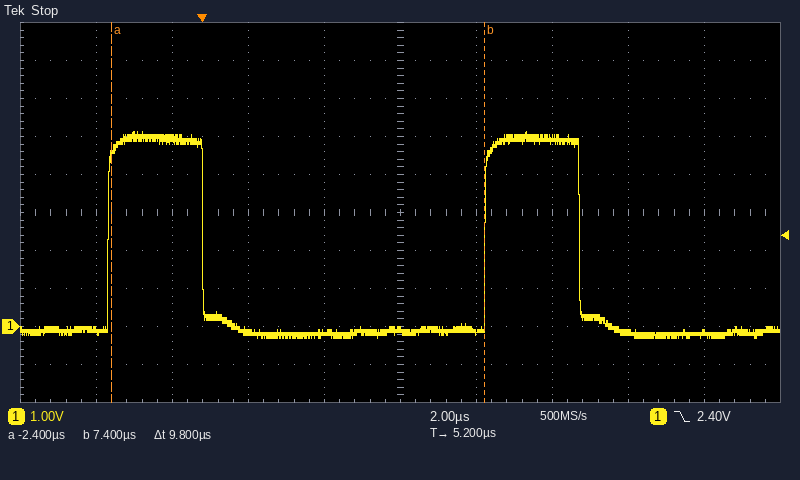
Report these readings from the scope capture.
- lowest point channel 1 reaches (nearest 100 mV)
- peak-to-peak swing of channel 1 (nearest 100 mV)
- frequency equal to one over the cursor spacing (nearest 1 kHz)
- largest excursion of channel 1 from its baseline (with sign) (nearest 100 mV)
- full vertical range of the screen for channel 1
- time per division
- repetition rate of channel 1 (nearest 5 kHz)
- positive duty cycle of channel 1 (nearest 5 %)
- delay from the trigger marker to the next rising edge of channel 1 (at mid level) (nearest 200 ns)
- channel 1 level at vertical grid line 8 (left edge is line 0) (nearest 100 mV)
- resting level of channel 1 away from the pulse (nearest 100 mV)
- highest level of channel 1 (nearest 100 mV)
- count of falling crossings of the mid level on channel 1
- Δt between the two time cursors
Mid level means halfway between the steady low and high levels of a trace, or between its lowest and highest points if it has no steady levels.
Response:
-300 mV
5.4 V
102 kHz
+5.3 V
10 V
2 µs
100 kHz
25 %
7.4 µs
-200 mV
-200 mV
5.1 V
2
9.8 µs
